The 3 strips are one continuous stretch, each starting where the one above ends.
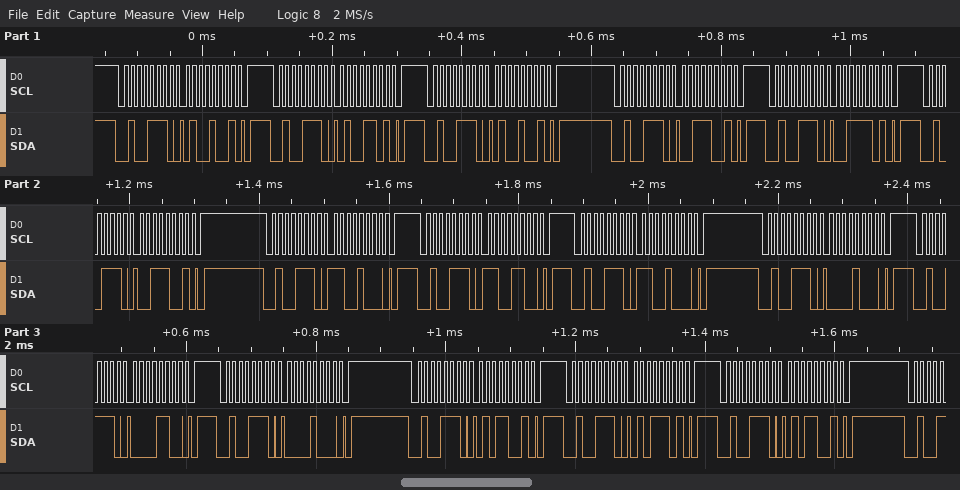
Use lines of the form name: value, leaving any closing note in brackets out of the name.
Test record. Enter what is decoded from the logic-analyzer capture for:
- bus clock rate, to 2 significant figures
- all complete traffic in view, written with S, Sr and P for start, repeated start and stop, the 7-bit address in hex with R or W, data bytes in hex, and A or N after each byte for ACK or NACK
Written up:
bus clock rate, to 2 significant figures: 100 kHz
all complete traffic in view, written with S, Sr and P for start, repeated start and stop, the 7-bit address in hex with R or W, data bytes in hex, and A or N after each byte for ACK or NACK: S 27W A 49 A P S 27W A 4D A P S 27W A 49 A P S 27W A 39 A P S 27W A 3D A P S 27W A 39 A P S 27W A C8 A P S 27W A CC A P S 27W A C8 A P S 27W A 08 A P S 27W A 0C A P S 27W A 08 A P S 27W A 59 A P S 27W A 5D A P S 27W A 59 A P
